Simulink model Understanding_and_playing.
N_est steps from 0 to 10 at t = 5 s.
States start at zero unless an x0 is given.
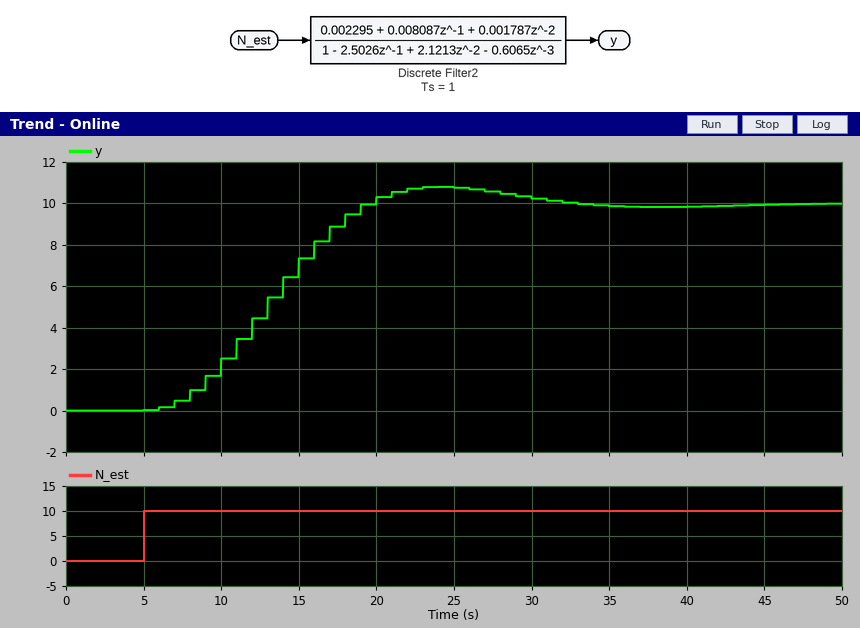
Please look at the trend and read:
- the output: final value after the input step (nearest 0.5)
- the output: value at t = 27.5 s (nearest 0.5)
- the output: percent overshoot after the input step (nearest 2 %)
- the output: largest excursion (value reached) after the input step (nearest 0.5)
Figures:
10.0
10.5
8 %
11.0
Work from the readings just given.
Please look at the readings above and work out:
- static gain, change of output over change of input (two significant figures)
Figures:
1.0
